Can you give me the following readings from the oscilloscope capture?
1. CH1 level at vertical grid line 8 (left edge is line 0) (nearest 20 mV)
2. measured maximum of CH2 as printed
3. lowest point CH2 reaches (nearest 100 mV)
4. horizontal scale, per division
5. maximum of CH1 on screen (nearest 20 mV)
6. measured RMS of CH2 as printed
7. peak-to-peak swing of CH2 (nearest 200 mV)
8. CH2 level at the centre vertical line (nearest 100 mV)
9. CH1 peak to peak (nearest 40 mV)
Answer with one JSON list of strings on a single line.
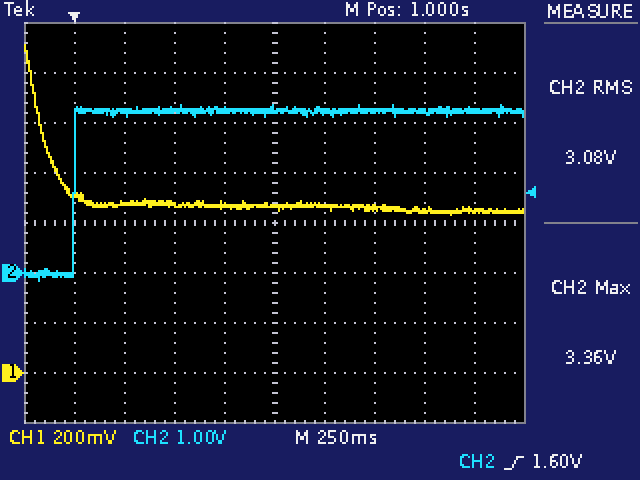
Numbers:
["640 mV", "3.36 V", "-200 mV", "250 ms", "1.32 V", "3.08 V", "3.6 V", "3.3 V", "680 mV"]
